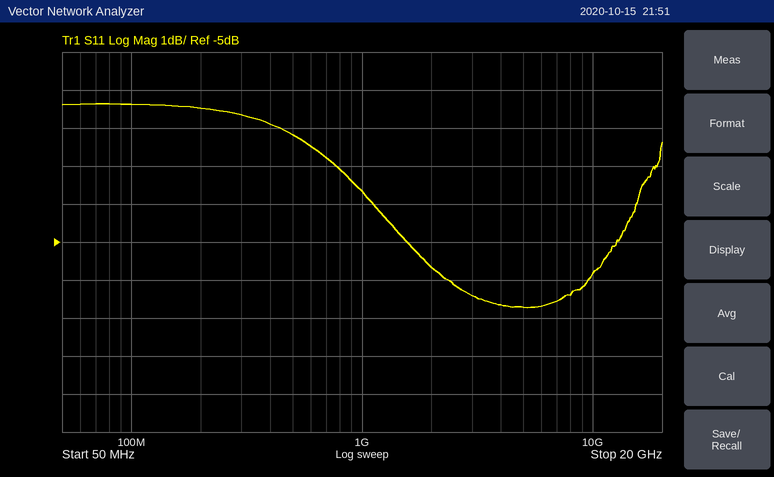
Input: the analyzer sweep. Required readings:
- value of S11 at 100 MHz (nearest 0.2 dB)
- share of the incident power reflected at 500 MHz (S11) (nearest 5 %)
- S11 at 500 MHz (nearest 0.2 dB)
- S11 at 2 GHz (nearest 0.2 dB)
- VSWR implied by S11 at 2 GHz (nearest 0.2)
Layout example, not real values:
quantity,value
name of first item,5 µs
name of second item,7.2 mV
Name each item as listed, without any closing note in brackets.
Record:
quantity,value
value of S11 at 100 MHz,-1.4 dB
share of the incident power reflected at 500 MHz (S11),60 %
S11 at 500 MHz,-2.2 dB
S11 at 2 GHz,-5.6 dB
VSWR implied by S11 at 2 GHz,3.2
